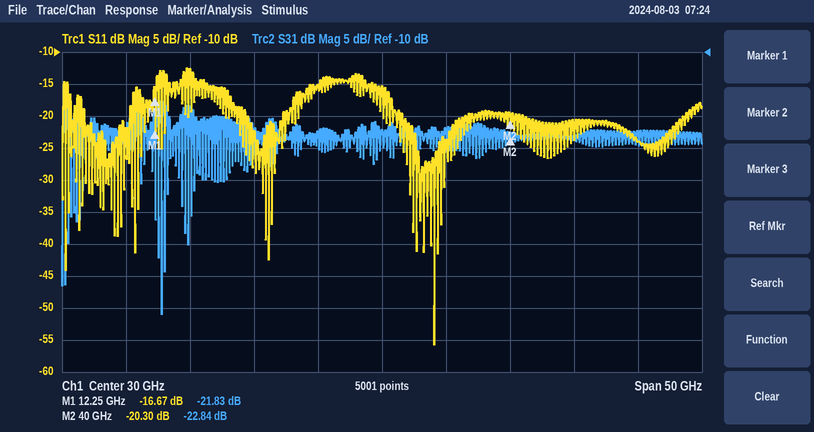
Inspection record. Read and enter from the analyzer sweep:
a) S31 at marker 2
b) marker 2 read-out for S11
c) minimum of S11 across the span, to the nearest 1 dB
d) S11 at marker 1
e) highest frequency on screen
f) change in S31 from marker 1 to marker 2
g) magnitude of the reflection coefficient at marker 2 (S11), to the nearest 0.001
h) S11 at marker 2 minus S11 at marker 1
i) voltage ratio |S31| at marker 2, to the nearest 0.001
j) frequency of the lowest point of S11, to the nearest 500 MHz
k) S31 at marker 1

-22.84 dB
-20.30 dB
-56 dB
-16.67 dB
55 GHz
-1.01 dB
0.097
-3.63 dB
0.072
34.0 GHz
-21.83 dB
